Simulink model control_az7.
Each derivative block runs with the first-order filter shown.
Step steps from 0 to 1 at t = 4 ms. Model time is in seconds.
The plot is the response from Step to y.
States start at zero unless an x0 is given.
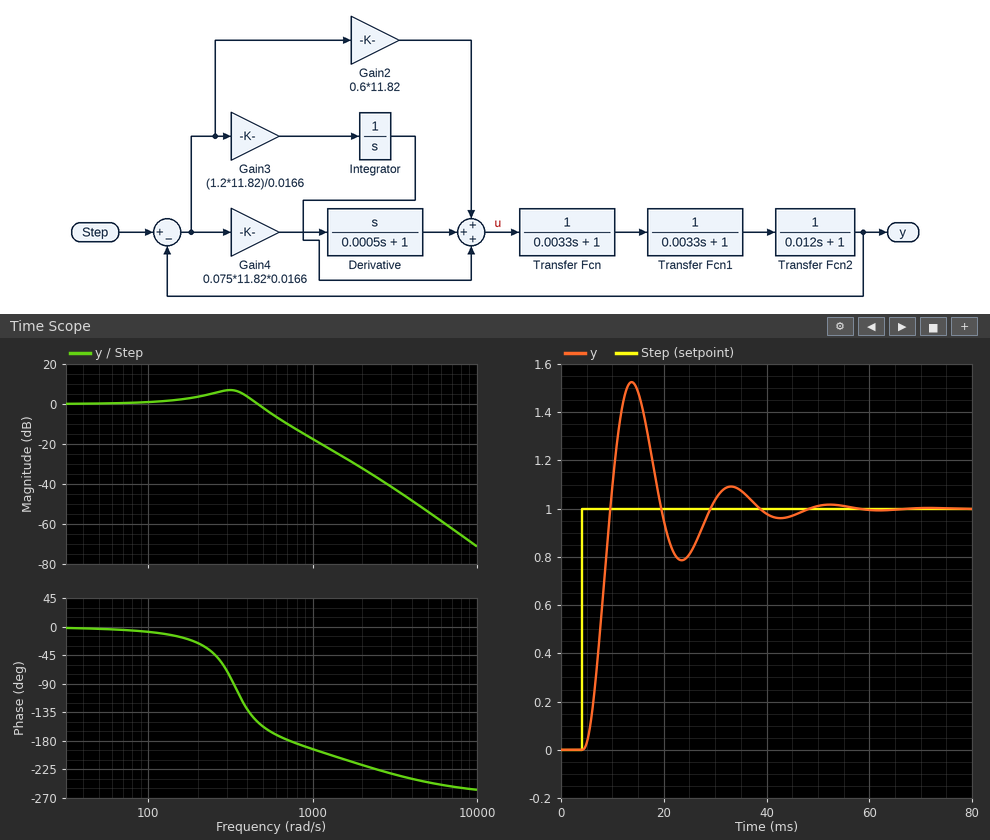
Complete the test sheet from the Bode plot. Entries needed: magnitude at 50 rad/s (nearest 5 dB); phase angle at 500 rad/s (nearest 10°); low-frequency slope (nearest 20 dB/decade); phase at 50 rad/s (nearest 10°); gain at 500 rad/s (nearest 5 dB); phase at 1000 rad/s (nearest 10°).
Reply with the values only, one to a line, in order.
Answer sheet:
0 dB
-160°
0 dB/decade
0°
0 dB
-190°
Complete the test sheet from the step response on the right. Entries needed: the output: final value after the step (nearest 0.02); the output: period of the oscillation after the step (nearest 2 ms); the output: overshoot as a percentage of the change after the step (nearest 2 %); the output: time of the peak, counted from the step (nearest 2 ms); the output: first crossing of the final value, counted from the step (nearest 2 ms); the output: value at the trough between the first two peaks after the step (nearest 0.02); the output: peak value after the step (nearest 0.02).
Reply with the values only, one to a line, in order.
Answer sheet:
1.00
20 ms
52 %
10 ms
6 ms
0.78
1.52
